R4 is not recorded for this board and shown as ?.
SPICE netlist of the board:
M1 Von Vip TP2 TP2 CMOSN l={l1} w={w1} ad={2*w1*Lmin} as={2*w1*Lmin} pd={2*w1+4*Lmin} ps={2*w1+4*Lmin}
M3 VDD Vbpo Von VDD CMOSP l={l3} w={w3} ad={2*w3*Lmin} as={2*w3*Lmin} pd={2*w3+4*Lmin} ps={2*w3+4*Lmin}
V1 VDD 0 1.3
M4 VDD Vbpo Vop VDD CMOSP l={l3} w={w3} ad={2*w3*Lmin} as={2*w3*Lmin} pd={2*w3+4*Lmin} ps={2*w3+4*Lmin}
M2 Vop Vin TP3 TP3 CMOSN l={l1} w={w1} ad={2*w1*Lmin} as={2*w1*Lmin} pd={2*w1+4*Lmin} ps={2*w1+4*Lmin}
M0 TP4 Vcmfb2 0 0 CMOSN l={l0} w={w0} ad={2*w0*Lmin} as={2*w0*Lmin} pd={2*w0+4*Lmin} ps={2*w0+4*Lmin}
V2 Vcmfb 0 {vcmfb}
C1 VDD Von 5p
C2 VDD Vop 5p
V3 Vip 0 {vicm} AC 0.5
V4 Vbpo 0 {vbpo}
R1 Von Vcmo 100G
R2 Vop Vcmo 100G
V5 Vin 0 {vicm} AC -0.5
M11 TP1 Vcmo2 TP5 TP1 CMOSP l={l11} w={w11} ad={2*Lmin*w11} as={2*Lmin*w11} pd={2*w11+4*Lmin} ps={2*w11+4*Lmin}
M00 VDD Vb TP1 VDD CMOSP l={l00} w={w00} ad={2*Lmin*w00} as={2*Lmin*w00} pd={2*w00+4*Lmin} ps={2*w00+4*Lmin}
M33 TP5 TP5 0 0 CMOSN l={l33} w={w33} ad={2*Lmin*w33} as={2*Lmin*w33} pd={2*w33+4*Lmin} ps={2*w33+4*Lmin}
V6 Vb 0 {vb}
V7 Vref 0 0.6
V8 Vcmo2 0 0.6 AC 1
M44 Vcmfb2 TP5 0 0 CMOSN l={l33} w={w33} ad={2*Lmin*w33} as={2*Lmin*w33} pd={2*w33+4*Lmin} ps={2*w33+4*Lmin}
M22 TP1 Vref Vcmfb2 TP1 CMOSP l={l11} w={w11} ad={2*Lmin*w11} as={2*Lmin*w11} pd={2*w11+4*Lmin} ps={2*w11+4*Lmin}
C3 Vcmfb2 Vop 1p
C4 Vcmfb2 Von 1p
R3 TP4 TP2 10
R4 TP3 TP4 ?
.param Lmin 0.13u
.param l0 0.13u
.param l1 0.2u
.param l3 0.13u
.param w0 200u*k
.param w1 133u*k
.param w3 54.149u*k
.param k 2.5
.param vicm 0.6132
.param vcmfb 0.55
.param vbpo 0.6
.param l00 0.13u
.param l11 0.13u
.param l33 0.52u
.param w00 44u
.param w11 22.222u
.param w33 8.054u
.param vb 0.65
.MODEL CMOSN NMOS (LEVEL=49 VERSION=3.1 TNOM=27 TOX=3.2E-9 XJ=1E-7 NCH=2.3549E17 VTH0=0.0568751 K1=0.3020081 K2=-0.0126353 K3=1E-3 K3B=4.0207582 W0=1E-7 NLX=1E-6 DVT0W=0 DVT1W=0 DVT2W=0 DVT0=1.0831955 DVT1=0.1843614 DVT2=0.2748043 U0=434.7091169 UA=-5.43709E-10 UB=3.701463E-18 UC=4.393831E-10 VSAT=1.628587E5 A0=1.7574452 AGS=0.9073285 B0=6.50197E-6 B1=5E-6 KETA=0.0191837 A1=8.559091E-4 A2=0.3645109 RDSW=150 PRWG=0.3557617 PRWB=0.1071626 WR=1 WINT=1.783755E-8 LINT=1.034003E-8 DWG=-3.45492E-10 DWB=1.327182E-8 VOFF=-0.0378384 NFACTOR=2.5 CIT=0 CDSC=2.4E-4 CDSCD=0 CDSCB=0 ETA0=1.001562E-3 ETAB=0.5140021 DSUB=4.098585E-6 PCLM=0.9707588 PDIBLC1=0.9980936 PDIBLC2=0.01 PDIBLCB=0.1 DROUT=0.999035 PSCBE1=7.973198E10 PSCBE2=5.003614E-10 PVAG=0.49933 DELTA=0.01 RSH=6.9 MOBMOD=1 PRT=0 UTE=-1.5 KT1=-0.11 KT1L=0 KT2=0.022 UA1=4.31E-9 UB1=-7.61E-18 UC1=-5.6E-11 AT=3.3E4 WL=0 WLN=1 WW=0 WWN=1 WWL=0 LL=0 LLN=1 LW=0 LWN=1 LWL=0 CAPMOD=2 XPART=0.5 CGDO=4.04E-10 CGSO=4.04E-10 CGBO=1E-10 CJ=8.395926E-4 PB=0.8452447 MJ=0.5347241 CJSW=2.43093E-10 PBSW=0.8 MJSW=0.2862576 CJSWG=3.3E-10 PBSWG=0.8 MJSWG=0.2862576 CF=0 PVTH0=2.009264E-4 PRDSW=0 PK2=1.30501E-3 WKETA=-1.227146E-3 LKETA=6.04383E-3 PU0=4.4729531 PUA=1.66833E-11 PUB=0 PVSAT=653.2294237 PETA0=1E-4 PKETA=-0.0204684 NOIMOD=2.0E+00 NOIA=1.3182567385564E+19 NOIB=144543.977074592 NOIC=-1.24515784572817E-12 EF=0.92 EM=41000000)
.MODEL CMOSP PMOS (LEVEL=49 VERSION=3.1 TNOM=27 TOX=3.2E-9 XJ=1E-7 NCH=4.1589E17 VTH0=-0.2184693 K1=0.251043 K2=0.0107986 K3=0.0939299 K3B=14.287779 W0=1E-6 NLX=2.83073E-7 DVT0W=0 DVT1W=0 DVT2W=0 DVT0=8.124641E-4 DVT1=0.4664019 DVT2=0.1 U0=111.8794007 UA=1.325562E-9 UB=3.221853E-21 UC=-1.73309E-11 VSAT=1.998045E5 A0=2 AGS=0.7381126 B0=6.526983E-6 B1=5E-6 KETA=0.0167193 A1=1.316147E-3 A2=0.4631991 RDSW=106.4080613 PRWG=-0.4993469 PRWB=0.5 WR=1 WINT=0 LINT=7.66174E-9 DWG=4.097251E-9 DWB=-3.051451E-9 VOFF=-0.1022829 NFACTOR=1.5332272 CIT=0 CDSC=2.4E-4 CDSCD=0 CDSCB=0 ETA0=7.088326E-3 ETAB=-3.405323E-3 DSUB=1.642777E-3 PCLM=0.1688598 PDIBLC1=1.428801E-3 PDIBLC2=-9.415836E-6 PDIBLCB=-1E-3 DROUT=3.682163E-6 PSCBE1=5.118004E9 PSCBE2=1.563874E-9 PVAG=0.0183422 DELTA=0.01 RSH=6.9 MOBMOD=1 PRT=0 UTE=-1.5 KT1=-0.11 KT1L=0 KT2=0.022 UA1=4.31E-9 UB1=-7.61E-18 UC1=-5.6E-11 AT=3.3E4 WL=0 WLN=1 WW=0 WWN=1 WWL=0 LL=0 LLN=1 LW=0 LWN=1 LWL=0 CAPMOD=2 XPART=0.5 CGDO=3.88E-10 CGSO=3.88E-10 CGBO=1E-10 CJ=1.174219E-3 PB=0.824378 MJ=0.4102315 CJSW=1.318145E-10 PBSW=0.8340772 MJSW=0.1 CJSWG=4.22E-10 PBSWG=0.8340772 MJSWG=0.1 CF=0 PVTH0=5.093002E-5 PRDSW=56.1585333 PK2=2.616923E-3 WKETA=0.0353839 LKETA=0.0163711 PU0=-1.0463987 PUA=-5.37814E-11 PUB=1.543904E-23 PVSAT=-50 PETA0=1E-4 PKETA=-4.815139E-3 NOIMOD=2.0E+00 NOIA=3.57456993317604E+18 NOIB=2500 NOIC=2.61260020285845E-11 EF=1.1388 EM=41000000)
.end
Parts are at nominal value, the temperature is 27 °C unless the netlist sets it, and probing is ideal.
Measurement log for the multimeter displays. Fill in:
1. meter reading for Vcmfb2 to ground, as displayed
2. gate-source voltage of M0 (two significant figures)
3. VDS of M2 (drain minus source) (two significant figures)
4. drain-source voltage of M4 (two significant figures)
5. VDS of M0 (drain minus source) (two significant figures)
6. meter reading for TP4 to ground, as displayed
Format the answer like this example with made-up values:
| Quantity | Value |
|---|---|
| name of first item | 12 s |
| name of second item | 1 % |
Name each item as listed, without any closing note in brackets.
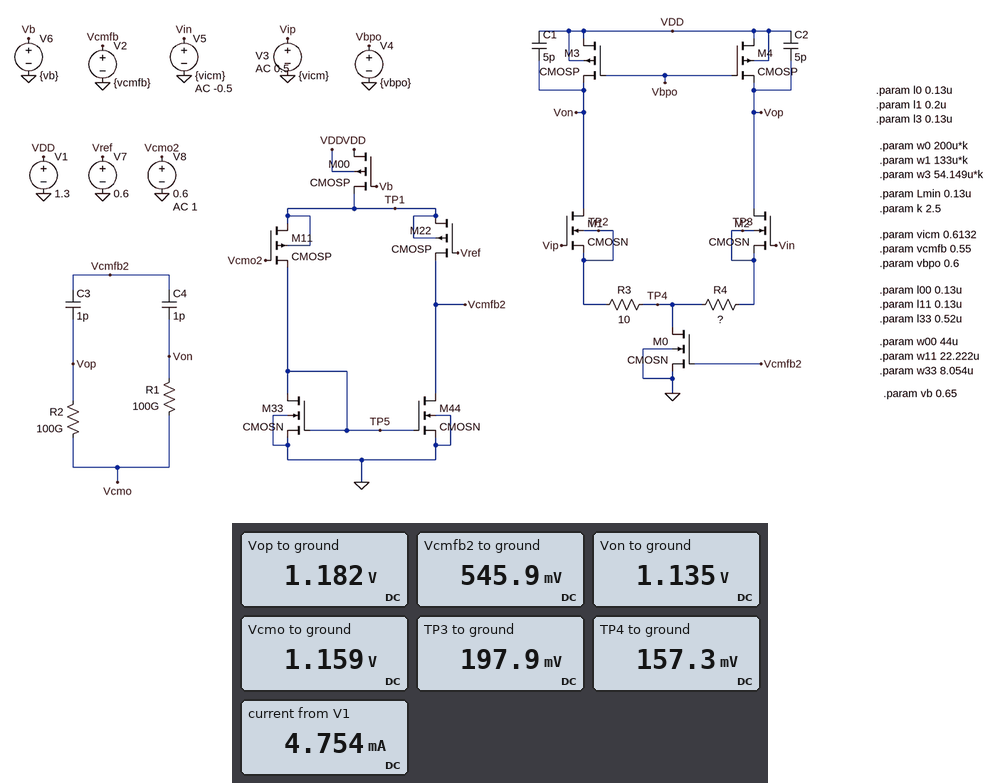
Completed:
| Quantity | Value |
|---|---|
| meter reading for Vcmfb2 to ground, as displayed | 545.9 mV |
| gate-source voltage of M0 | 550 mV |
| VDS of M2 (drain minus source) | 980 mV |
| drain-source voltage of M4 | 120 mV |
| VDS of M0 (drain minus source) | 160 mV |
| meter reading for TP4 to ground, as displayed | 157.3 mV |
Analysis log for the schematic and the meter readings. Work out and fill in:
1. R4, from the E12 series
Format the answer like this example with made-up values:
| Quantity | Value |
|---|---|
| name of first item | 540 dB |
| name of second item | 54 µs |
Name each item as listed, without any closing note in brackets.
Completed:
| Quantity | Value |
|---|---|
| R4, from the E12 series | 22 Ω |
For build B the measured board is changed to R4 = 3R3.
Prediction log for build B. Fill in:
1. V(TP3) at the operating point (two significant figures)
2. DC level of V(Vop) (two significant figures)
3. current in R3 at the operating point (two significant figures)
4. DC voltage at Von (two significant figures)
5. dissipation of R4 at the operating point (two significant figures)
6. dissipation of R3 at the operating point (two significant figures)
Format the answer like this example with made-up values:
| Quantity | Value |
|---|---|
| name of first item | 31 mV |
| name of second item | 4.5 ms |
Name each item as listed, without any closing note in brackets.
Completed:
| Quantity | Value |
|---|---|
| V(TP3) at the operating point | 180 mV |
| DC level of V(Vop) | 1.1 V |
| current in R3 at the operating point | 2.0 mA |
| DC voltage at Von | 1.2 V |
| dissipation of R4 at the operating point | 18 µW |
| dissipation of R3 at the operating point | 39 µW |
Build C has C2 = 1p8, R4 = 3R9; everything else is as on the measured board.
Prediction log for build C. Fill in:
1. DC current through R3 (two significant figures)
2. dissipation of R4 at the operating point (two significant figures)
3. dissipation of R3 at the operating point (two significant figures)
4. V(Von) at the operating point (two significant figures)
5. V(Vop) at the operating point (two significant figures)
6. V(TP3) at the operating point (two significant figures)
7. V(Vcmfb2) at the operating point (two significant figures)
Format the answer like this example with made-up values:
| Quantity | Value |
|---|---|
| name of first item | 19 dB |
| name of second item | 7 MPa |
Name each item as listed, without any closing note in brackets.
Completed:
| Quantity | Value |
|---|---|
| DC current through R3 | 2.0 mA |
| dissipation of R4 at the operating point | 21 µW |
| dissipation of R3 at the operating point | 40 µW |
| V(Von) at the operating point | 1.2 V |
| V(Vop) at the operating point | 1.1 V |
| V(TP3) at the operating point | 180 mV |
| V(Vcmfb2) at the operating point | 550 mV |
